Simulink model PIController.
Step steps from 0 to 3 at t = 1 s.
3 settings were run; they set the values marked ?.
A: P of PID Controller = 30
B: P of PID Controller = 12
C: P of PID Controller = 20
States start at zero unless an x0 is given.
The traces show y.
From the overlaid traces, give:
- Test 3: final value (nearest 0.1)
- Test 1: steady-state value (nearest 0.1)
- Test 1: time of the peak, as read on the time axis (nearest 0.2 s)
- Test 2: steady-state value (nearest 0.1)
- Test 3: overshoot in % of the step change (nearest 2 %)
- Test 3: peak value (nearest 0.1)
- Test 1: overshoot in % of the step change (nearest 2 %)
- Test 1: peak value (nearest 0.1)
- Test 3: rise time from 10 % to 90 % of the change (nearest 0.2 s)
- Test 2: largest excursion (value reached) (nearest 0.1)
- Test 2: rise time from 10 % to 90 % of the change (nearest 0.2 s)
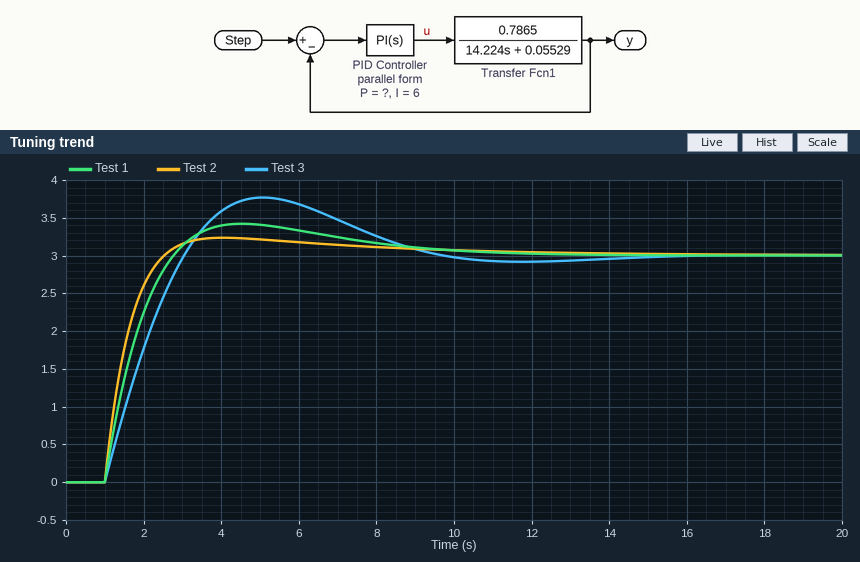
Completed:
3.0
3.0
4.6 s
3.0
26 %
3.8
14 %
3.4
1.6 s
3.2
1.0 s
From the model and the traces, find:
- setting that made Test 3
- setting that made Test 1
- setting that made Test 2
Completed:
B
C
A
